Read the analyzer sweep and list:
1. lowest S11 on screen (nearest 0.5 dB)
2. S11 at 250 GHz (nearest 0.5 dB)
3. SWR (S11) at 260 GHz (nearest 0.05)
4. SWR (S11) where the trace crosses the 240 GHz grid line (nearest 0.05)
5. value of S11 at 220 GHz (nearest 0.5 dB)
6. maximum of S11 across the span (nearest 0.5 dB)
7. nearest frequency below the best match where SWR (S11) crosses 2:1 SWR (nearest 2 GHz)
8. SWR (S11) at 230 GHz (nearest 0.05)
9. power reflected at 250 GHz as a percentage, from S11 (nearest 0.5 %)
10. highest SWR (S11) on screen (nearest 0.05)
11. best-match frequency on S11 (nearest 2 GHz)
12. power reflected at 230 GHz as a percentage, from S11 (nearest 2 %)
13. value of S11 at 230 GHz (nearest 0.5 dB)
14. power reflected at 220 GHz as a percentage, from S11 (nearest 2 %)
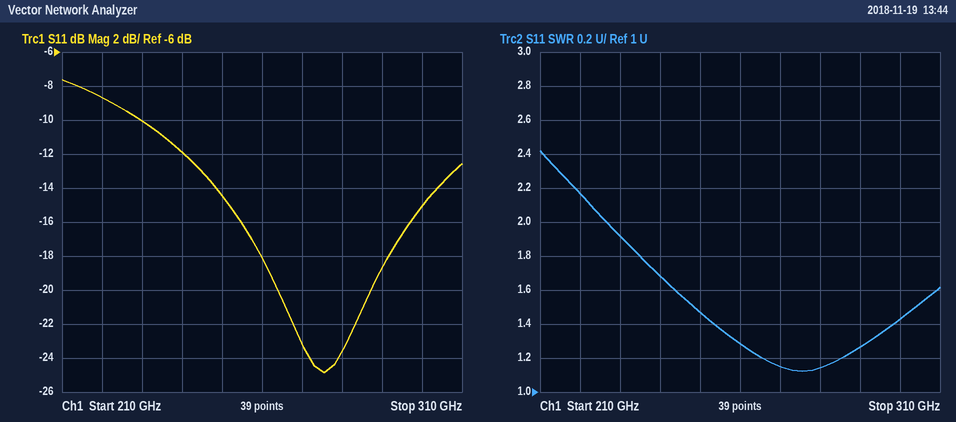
-25.0 dB
-14.5 dB
1.30
1.70
-8.5 dB
-7.5 dB
226 GHz
1.90
3.5 %
2.40
276 GHz
10 %
-10.0 dB
14 %
